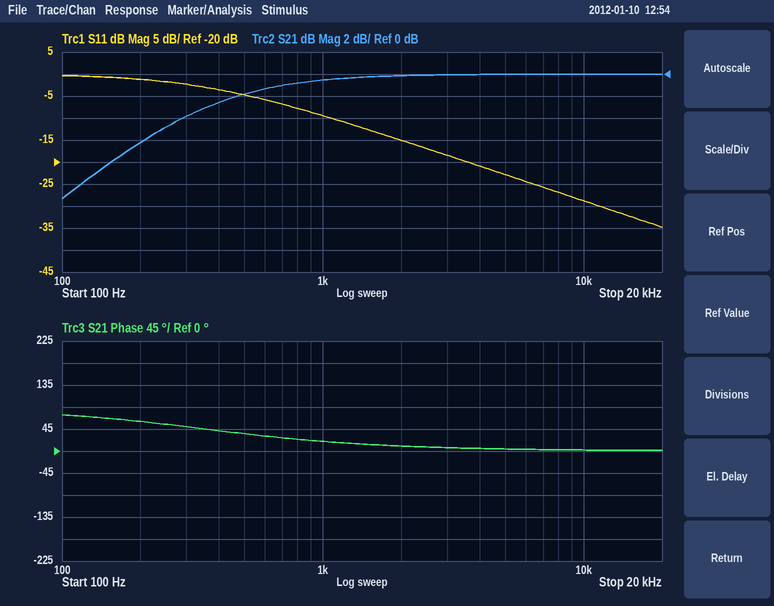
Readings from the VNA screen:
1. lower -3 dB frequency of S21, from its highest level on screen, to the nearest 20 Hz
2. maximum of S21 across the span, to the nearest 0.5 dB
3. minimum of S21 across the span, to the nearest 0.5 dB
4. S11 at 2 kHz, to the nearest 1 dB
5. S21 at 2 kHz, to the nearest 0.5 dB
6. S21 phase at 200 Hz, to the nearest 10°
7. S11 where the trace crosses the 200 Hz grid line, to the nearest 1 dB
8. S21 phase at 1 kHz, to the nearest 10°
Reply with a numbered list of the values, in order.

1. 360 Hz
2. 0.0 dB
3. -11.5 dB
4. -15 dB
5. 0.0 dB
6. 60°
7. -1 dB
8. 20°
